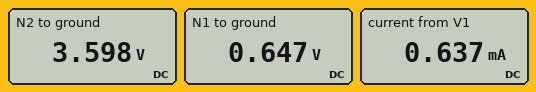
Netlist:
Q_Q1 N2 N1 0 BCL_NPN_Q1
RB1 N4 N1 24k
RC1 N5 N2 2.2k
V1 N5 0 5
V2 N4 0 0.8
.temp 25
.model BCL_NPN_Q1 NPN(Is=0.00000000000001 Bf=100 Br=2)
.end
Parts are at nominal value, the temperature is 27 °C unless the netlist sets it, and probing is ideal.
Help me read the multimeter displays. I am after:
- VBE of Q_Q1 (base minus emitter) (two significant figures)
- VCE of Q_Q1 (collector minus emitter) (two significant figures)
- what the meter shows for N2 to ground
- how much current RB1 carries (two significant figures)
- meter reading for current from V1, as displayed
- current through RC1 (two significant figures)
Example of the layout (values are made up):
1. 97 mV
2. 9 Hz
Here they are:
1. 650 mV
2. 3.6 V
3. 3.598 V
4. 6.4 µA
5. 0.637 mA
6. 640 µA
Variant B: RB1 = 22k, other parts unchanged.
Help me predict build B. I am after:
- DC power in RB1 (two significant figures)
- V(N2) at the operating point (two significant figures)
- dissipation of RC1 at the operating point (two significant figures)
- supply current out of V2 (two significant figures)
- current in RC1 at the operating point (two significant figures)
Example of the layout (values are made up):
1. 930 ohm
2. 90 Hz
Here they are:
1. 1.0 µW
2. 3.5 V
3. 1.0 mW
4. 6.9 µA
5. 690 µA
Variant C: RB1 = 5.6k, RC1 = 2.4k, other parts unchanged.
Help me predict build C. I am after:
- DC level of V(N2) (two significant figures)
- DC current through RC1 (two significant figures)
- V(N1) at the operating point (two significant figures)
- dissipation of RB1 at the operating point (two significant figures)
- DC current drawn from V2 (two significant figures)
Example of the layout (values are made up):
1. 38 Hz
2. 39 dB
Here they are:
1. 160 mV
2. 2.0 mA
3. 680 mV
4. 2.7 µW
5. 22 µA
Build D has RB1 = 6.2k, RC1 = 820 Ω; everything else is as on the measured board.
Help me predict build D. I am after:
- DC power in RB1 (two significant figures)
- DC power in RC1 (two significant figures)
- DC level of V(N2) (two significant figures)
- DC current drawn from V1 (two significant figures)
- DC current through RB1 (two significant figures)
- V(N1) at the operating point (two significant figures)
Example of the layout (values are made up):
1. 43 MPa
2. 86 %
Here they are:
1. 2.5 µW
2. 3.3 mW
3. 3.4 V
4. 2.0 mA
5. 20 µA
6. 680 mV
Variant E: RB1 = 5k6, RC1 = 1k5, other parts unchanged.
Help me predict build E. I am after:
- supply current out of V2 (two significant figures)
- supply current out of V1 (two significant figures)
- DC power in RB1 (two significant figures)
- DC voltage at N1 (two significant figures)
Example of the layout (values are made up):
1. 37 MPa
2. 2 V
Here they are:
1. 22 µA
2. 2.2 mA
3. 2.6 µW
4. 680 mV
